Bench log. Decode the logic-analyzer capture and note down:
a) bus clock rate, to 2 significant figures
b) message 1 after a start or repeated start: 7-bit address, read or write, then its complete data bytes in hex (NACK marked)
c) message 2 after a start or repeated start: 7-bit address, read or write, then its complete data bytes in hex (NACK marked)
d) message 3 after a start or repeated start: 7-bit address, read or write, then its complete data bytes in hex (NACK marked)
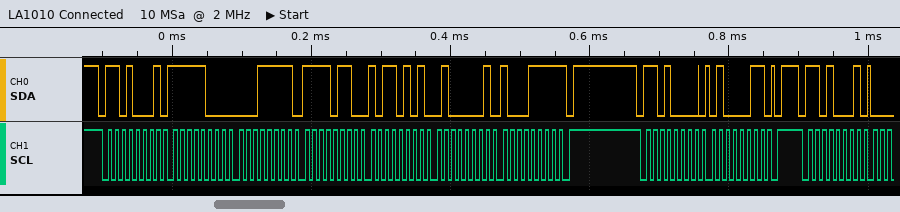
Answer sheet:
100 kHz
0x68 read: F8 1F F6 B5 41 8F NACK
0x68 write: 43
0x68 read
